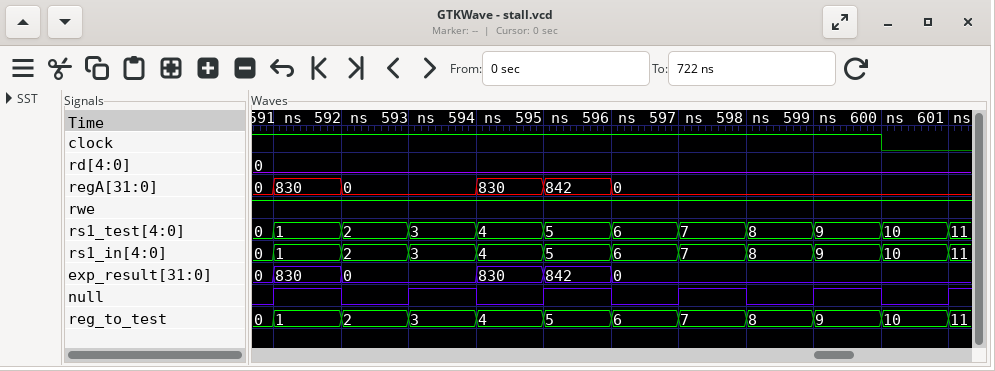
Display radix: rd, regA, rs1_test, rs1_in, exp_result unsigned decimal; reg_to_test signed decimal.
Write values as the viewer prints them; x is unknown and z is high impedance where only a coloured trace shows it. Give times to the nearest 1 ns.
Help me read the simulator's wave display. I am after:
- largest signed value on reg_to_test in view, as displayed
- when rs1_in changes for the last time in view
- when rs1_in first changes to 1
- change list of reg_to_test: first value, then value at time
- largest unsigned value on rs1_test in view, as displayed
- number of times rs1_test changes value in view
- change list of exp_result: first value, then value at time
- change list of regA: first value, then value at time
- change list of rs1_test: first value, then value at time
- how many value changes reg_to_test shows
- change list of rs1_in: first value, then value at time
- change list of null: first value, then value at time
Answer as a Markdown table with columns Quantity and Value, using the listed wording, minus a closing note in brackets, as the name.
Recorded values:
| Quantity | Value |
|---|---|
| largest signed value on reg_to_test in view, as displayed | 11 |
| when rs1_in changes for the last time in view | 601 ns |
| when rs1_in first changes to 1 | 591 ns |
| change list of reg_to_test: first value, then value at time | 0, 1 at 591 ns, 2 at 592 ns, 3 at 593 ns, 4 at 594 ns, 5 at 595 ns, 6 at 596 ns, 7 at 597 ns, 8 at 598 ns, 9 at 599 ns, 10 at 600 ns, 11 at 601 ns |
| largest unsigned value on rs1_test in view, as displayed | 11 |
| number of times rs1_test changes value in view | 11 |
| change list of exp_result: first value, then value at time | 0, 830 at 591 ns, 0 at 592 ns, 830 at 594 ns, 842 at 595 ns, 0 at 596 ns |
| change list of regA: first value, then value at time | 0, 830 at 591 ns, 0 at 592 ns, 830 at 594 ns, 842 at 595 ns, 0 at 596 ns |
| change list of rs1_test: first value, then value at time | 0, 1 at 591 ns, 2 at 592 ns, 3 at 593 ns, 4 at 594 ns, 5 at 595 ns, 6 at 596 ns, 7 at 597 ns, 8 at 598 ns, 9 at 599 ns, 10 at 600 ns, 11 at 601 ns |
| how many value changes reg_to_test shows | 11 |
| change list of rs1_in: first value, then value at time | 0, 1 at 591 ns, 2 at 592 ns, 3 at 593 ns, 4 at 594 ns, 5 at 595 ns, 6 at 596 ns, 7 at 597 ns, 8 at 598 ns, 9 at 599 ns, 10 at 600 ns, 11 at 601 ns |
| change list of null: first value, then value at time | 0, 1 at 591 ns, 0 at 592 ns, 1 at 593 ns, 0 at 594 ns, 1 at 595 ns, 0 at 596 ns, 1 at 597 ns, 0 at 598 ns, 1 at 599 ns, 0 at 600 ns, 1 at 601 ns |
